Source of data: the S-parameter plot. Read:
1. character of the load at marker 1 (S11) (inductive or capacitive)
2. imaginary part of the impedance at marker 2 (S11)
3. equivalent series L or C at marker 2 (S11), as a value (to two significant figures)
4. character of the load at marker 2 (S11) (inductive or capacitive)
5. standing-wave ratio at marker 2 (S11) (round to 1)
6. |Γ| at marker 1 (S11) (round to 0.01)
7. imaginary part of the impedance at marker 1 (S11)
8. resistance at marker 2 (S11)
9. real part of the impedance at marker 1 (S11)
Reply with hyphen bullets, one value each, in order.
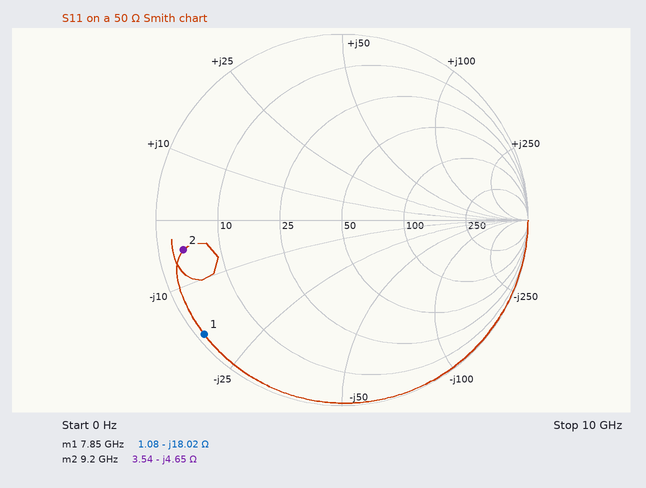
- capacitive
- -4.65 Ω
- 3.7 pF
- capacitive
- 14
- 0.96
- -18.02 Ω
- 3.54 Ω
- 1.08 Ω
